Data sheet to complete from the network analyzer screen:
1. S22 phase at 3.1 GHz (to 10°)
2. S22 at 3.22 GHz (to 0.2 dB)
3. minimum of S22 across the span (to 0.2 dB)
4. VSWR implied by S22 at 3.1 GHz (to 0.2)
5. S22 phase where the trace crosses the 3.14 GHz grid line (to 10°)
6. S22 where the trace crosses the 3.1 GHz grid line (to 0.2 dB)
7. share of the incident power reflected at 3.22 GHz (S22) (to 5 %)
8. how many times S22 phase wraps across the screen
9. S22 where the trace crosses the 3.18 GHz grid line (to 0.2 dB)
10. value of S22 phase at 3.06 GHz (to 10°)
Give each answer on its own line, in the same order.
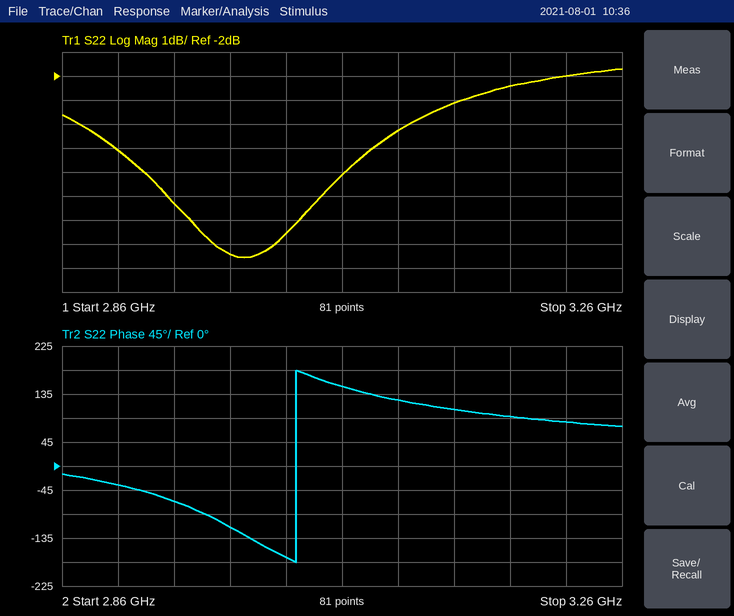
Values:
120°
-2.0 dB
-9.6 dB
4.2
110°
-4.2 dB
65 %
1
-2.4 dB
150°
